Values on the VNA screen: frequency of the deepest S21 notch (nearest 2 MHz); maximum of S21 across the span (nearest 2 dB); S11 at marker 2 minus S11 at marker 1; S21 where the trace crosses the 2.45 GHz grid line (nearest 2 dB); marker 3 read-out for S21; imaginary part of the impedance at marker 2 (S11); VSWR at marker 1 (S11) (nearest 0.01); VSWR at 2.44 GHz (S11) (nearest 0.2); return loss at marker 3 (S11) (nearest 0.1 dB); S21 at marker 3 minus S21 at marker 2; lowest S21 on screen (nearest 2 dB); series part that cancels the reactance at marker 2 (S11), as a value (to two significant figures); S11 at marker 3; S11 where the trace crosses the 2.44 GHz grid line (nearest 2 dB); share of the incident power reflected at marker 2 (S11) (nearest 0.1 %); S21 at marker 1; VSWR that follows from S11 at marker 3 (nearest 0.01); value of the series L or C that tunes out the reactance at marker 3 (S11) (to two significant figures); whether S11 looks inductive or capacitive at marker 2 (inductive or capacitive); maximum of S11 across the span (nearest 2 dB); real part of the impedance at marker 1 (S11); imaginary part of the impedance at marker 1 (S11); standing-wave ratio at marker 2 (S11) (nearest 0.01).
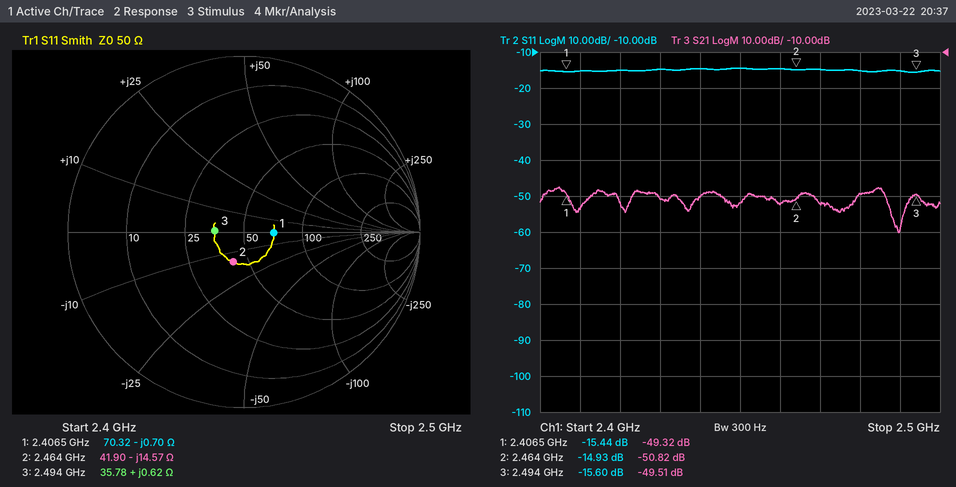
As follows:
2.490 GHz
-48 dB
0.51 dB
-52 dB
-49.51 dB
-14.57 Ω
1.41
1.4
15.6 dB
1.31 dB
-60 dB
940 pH
-15.60 dB
-14 dB
3.2 %
-49.32 dB
1.40
100 pF
capacitive
-14 dB
70.32 Ω
-0.70 Ω
1.44
